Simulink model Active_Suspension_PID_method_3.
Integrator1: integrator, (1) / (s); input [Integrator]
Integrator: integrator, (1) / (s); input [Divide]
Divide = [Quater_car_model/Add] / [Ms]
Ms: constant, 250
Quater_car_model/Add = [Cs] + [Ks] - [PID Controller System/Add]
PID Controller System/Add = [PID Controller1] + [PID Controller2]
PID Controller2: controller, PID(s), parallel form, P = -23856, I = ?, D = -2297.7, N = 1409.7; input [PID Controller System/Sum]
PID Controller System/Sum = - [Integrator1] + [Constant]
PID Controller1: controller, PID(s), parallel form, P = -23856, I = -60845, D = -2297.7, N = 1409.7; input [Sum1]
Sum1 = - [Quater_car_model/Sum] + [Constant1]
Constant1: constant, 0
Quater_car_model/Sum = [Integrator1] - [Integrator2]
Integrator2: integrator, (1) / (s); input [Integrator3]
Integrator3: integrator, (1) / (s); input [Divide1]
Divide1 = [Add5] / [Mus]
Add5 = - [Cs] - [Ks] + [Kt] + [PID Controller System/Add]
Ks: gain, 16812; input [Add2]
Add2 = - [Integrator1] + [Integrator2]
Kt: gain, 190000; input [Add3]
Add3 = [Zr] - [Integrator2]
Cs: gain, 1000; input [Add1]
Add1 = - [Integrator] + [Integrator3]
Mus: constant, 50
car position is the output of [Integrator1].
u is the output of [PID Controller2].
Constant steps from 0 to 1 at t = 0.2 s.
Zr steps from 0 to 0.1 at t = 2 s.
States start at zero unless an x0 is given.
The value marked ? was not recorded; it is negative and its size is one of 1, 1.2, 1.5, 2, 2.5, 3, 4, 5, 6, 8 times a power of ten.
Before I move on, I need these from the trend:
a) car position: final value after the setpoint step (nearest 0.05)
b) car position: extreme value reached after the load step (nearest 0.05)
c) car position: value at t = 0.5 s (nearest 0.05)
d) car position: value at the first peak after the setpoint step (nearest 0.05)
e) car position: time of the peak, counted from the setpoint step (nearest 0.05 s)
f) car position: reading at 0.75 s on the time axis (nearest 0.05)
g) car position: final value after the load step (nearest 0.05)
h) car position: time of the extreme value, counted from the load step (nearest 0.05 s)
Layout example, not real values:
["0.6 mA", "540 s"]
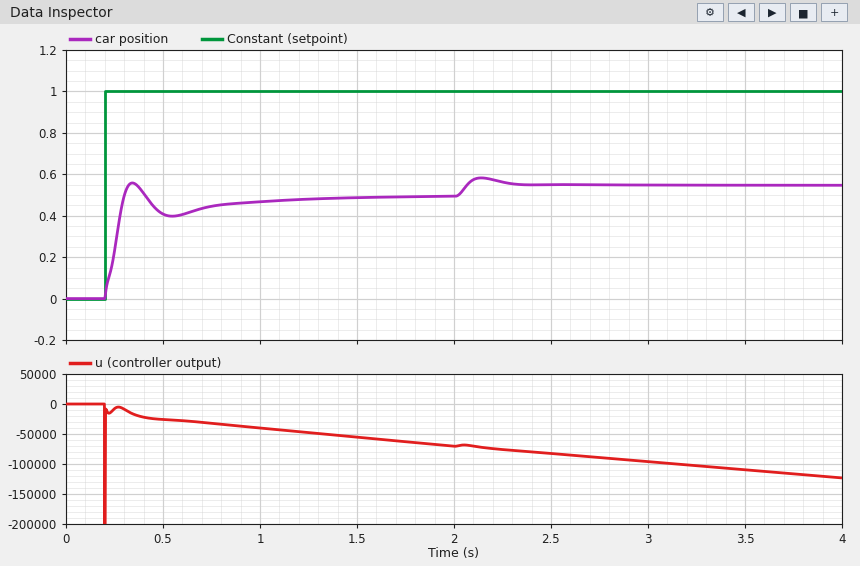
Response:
["0.50", "0.60", "0.40", "0.55", "0.15 s", "0.45", "0.55", "0.15 s"]
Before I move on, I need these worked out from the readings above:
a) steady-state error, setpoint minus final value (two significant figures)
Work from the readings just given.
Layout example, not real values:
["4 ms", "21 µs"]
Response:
["0.50"]
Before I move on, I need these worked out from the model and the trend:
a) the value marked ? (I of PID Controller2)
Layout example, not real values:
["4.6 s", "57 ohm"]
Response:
["-60000"]
